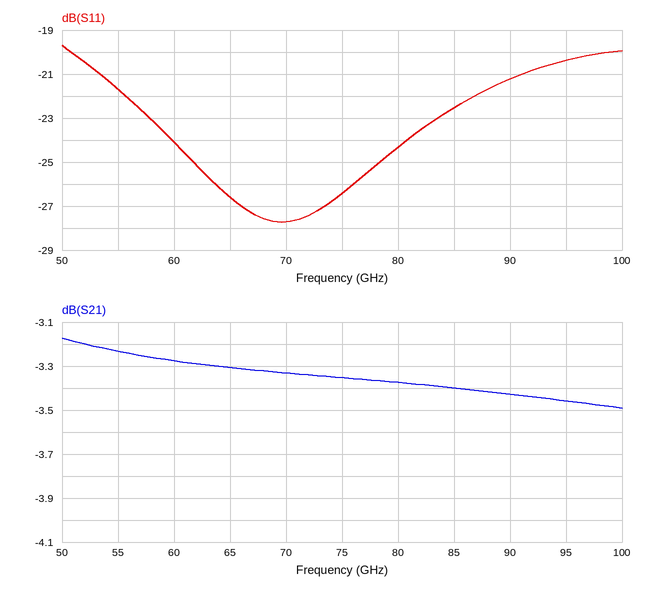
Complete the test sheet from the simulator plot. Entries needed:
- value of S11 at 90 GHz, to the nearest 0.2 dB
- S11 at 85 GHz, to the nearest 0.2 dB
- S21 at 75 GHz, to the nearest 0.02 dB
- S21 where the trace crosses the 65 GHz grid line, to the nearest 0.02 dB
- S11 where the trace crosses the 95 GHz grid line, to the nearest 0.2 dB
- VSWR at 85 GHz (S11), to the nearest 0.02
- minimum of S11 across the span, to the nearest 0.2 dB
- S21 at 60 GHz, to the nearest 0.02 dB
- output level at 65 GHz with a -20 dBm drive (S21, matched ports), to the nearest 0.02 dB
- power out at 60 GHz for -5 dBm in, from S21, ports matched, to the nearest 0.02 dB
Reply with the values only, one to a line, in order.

-21.2 dB
-22.6 dB
-3.36 dB
-3.30 dB
-20.4 dB
1.16
-27.8 dB
-3.28 dB
-23.30 dBm
-8.28 dBm
